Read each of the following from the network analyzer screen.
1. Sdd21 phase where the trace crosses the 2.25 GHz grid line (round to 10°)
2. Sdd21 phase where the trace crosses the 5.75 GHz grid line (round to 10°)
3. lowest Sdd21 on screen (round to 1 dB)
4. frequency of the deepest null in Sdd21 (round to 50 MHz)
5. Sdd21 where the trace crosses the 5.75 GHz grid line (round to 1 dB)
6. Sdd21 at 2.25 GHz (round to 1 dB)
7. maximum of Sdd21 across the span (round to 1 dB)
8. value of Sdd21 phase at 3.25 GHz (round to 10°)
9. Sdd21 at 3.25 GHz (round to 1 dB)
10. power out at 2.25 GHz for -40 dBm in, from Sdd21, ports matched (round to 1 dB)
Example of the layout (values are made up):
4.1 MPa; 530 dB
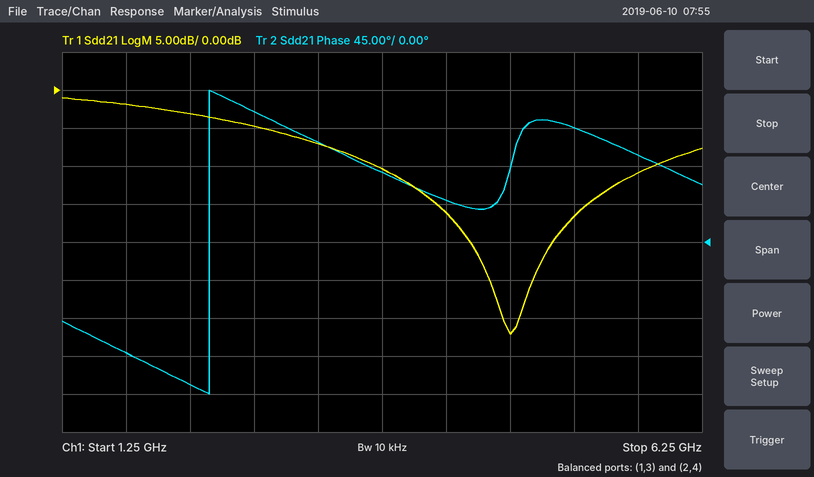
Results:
-170°; 100°; -32 dB; 4.75 GHz; -11 dB; -3 dB; -1 dB; 120°; -7 dB; -43 dBm
